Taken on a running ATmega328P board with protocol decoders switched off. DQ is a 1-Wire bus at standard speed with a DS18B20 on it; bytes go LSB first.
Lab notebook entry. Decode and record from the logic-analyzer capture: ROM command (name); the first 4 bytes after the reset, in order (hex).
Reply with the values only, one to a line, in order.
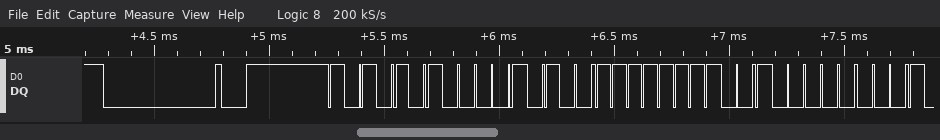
Match ROM
55 28 FF 04
